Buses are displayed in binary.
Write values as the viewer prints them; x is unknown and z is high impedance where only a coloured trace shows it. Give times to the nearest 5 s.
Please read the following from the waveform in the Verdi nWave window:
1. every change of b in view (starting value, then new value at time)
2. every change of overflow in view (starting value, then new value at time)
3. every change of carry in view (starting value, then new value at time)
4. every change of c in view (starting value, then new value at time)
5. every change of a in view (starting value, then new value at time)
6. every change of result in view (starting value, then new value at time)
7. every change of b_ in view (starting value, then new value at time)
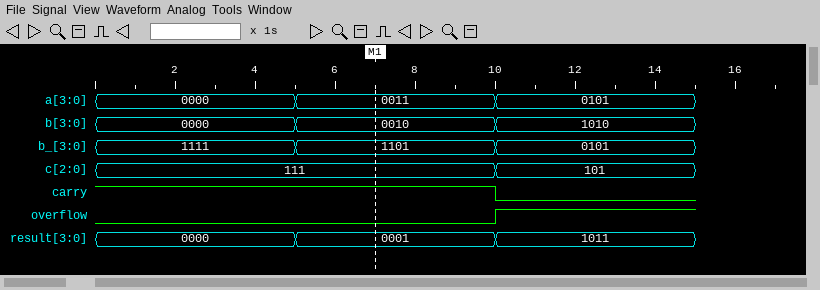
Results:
0000, 0010 at 5 s, 1010 at 10 s
0, 1 at 10 s
1, 0 at 10 s
111, 101 at 10 s
0000, 0011 at 5 s, 0101 at 10 s
0000, 0001 at 5 s, 1011 at 10 s
1111, 1101 at 5 s, 0101 at 10 s
